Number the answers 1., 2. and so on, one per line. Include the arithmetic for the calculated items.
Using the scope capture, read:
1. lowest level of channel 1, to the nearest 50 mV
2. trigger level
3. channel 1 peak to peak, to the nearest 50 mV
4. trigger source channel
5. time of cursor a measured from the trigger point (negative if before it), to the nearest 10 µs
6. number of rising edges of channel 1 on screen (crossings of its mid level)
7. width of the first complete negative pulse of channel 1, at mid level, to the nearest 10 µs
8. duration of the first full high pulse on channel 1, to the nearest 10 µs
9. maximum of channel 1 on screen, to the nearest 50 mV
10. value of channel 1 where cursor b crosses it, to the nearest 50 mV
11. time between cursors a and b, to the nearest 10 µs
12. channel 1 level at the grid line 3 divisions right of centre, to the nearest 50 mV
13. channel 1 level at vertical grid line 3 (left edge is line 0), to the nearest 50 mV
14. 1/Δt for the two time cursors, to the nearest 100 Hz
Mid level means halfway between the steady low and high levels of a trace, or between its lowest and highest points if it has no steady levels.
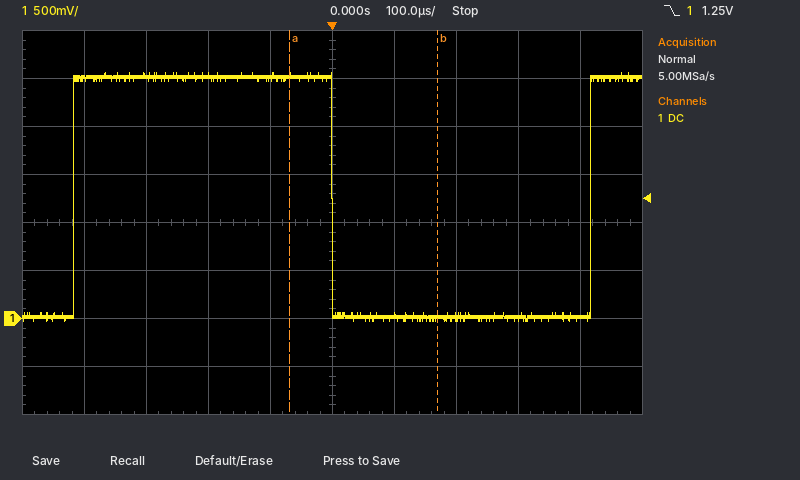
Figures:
1. -50 mV
2. 1.25 V
3. 2.55 V − (-50 mV) = 2.60 V
4. channel 1
5. -70 µs
6. 2
7. 420 µs
8. 420 µs
9. 2.55 V
10. 0 mV
11. 240 µs
12. 0 mV
13. 2.55 V
14. 1 / 240 µs ≈ 4.2 kHz
